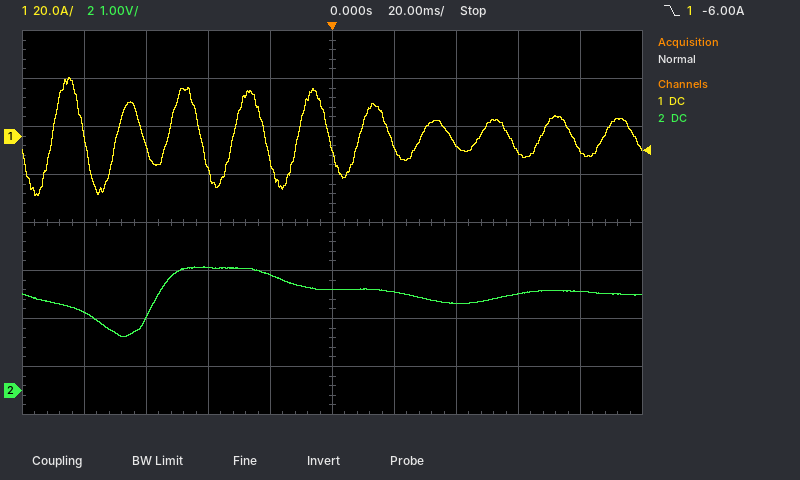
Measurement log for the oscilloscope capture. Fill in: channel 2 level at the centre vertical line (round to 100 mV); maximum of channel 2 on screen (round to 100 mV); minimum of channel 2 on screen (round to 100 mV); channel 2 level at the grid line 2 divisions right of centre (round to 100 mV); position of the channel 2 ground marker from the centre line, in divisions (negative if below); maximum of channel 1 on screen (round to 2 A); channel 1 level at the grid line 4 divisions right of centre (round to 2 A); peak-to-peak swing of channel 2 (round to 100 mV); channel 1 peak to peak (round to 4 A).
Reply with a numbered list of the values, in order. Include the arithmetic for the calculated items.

1. 2.1 V
2. 2.6 V
3. 1.1 V
4. 1.8 V
5. -3.5 div
6. 24 A
7. -6 A
8. 2.6 V − (1.1 V) = 1.5 V
9. 48 A
